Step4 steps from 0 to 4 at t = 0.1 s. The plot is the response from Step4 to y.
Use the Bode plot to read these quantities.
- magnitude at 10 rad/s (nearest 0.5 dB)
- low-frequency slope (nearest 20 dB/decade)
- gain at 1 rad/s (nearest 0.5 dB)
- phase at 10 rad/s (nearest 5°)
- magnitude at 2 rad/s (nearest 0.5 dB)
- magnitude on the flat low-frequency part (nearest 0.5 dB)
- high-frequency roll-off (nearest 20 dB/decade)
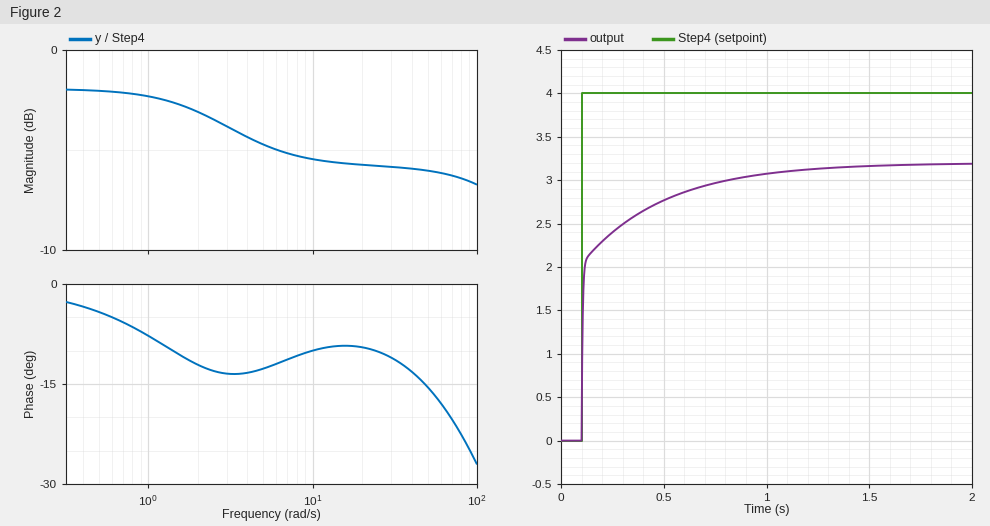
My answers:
-5.5 dB
0 dB/decade
-2.5 dB
-10°
-3.0 dB
-2.0 dB
0 dB/decade
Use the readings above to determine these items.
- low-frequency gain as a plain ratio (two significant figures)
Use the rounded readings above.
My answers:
0.79
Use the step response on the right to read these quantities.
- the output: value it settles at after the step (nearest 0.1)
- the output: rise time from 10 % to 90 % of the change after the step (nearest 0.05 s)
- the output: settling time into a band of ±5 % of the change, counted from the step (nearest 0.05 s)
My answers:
3.2
0.50 s
0.80 s
